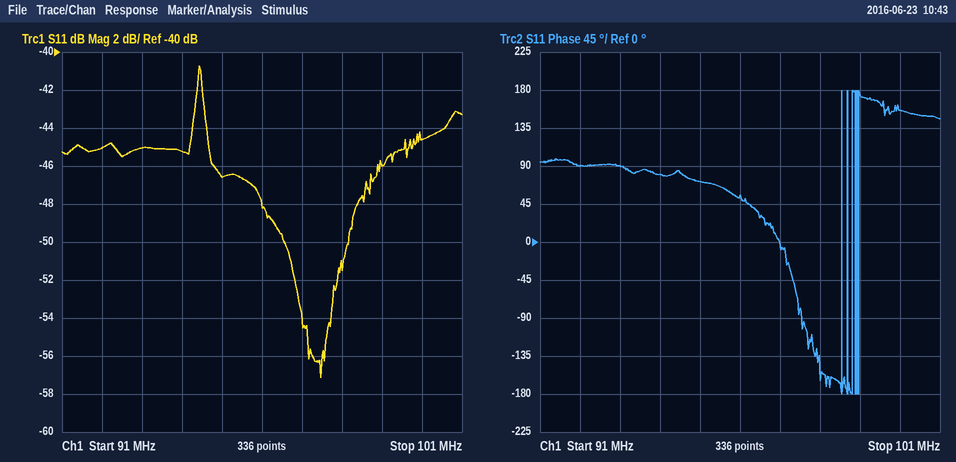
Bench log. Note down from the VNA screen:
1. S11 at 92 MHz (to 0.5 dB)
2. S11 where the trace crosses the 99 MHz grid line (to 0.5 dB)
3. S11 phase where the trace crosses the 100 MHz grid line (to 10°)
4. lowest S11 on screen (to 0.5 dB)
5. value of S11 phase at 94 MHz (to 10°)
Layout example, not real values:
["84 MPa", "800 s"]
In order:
["-45.0 dB", "-46.0 dB", "160°", "-57.0 dB", "80°"]
